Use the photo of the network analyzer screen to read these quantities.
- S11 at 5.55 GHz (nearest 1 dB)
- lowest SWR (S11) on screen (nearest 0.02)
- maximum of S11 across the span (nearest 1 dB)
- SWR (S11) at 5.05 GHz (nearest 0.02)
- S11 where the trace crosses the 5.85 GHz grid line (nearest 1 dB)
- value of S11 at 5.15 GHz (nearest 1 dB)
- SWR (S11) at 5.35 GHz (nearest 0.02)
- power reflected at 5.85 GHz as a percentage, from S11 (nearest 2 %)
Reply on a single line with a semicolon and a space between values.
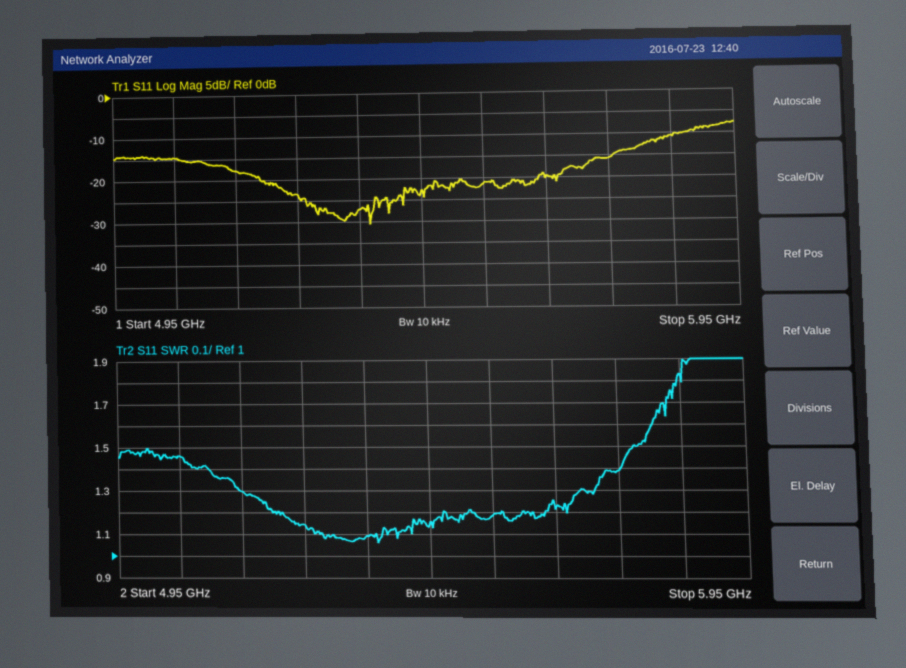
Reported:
-21 dB; 1.06; -8 dB; 1.46; -11 dB; -18 dB; 1.10; 8 %
